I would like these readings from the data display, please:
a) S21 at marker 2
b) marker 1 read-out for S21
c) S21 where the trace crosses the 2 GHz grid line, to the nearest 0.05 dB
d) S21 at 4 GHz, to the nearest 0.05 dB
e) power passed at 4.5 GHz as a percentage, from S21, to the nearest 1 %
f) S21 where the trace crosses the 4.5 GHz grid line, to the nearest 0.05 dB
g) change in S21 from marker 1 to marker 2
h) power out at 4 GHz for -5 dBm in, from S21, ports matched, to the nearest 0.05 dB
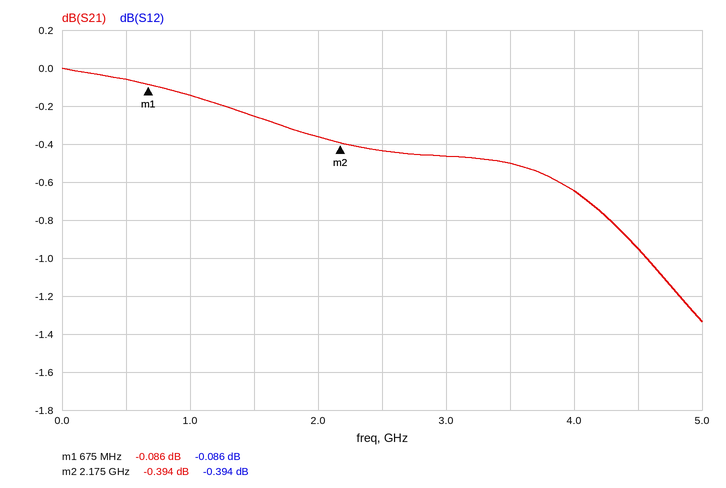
-0.394 dB
-0.086 dB
-0.35 dB
-0.65 dB
80 %
-0.95 dB
-0.308 dB
-5.65 dBm
